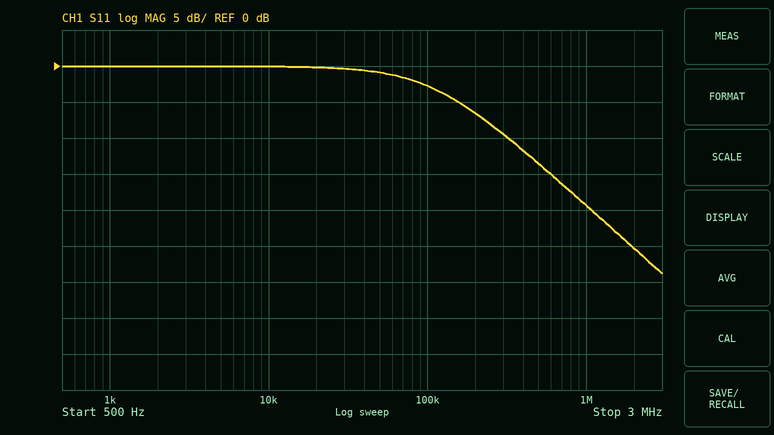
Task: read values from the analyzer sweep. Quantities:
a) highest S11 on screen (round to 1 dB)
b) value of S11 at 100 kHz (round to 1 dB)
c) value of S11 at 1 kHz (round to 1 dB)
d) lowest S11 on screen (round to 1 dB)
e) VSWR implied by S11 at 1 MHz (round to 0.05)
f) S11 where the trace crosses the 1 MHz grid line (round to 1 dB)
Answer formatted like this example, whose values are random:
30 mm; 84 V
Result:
0 dB; -3 dB; 0 dB; -29 dB; 1.25; -19 dB
